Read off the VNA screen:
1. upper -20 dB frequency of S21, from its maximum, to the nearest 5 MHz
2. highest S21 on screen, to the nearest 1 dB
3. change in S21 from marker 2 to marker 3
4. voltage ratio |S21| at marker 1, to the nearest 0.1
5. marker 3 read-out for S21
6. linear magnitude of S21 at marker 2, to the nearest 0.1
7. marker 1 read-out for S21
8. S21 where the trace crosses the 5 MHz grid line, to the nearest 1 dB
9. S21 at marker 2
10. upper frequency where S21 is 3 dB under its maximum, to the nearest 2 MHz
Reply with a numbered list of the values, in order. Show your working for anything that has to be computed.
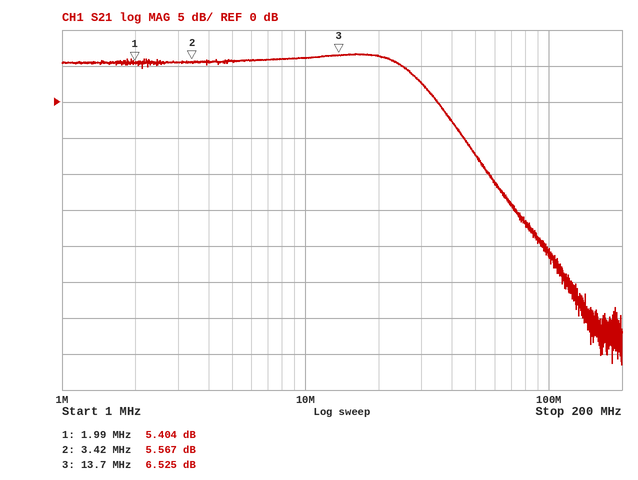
1. 65 MHz
2. 7 dB
3. 6.525 − (5.567) = 0.958 dB
4. 10^(5.404/20) ≈ 1.9
5. 6.525 dB
6. 10^(5.567/20) ≈ 1.9
7. 5.404 dB
8. 6 dB
9. 5.567 dB
10. 28 MHz
